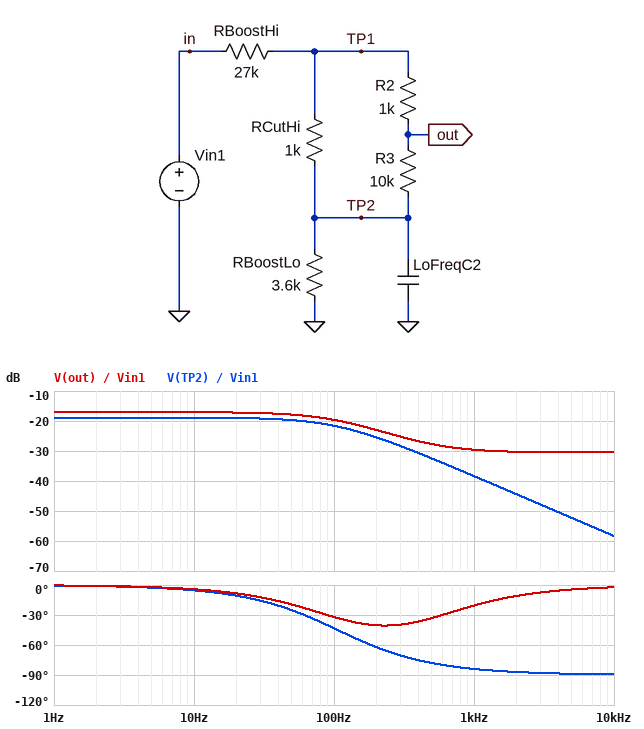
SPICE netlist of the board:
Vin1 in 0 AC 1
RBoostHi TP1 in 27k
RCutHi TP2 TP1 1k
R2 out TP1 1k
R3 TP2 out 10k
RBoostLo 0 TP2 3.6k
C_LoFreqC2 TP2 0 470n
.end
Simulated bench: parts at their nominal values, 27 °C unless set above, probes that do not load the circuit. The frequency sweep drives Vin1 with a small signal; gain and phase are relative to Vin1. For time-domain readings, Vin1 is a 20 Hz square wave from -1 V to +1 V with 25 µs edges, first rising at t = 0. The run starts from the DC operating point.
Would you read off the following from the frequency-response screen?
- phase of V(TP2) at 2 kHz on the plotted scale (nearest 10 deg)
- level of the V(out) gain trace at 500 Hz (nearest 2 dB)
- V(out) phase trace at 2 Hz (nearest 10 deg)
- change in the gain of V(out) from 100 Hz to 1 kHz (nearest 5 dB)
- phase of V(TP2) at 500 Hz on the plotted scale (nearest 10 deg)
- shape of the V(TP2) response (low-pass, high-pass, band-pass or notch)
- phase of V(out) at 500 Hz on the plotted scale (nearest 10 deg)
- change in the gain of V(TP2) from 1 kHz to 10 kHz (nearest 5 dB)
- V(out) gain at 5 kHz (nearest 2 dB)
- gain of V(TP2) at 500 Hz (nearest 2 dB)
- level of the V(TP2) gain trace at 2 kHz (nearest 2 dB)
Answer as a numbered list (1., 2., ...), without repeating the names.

1. -90 deg
2. -28 dB
3. 0 deg
4. -10 dB
5. -80 deg
6. low-pass
7. -30 deg
8. -20 dB
9. -30 dB
10. -32 dB
11. -44 dB
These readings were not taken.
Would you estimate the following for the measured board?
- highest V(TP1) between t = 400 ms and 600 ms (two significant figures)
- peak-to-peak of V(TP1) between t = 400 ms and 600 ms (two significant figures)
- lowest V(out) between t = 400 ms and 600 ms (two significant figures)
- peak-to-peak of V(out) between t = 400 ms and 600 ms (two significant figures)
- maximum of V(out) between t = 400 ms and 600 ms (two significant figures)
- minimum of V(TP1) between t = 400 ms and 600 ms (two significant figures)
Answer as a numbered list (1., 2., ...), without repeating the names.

1. 140 mV
2. 290 mV
3. -140 mV
4. 280 mV
5. 140 mV
6. -140 mV
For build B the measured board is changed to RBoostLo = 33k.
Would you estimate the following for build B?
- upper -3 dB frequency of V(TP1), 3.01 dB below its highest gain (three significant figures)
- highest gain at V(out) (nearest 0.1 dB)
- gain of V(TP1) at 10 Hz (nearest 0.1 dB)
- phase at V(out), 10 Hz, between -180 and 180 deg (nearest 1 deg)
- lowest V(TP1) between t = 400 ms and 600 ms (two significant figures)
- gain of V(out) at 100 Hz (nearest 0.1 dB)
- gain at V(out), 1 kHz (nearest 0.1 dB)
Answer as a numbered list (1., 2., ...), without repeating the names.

1. 22.5 Hz
2. -5.1 dB
3. -5.9 dB
4. -23 deg
5. -530 mV
6. -18.1 dB
7. -29.8 dB
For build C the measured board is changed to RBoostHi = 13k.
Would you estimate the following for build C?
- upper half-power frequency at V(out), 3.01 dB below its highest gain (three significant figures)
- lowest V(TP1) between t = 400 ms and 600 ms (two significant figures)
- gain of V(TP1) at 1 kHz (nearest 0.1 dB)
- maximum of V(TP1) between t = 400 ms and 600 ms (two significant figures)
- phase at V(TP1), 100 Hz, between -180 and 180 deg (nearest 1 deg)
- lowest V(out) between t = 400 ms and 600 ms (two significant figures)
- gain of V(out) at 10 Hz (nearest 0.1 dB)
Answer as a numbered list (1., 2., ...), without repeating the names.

1. 126 Hz
2. -260 mV
3. -22.8 dB
4. 260 mV
5. -28 deg
6. -250 mV
7. -12.0 dB
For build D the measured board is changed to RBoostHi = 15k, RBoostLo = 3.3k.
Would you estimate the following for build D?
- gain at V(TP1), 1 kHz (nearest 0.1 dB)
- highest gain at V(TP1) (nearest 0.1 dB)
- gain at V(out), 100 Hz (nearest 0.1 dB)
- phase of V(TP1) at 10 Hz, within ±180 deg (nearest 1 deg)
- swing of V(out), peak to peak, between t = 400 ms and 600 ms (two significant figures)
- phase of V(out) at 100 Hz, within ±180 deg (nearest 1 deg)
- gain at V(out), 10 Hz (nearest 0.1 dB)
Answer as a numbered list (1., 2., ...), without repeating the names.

1. -24.0 dB
2. -13.2 dB
3. -15.4 dB
4. -3 deg
5. 430 mV
6. -28 deg
7. -13.4 dB
